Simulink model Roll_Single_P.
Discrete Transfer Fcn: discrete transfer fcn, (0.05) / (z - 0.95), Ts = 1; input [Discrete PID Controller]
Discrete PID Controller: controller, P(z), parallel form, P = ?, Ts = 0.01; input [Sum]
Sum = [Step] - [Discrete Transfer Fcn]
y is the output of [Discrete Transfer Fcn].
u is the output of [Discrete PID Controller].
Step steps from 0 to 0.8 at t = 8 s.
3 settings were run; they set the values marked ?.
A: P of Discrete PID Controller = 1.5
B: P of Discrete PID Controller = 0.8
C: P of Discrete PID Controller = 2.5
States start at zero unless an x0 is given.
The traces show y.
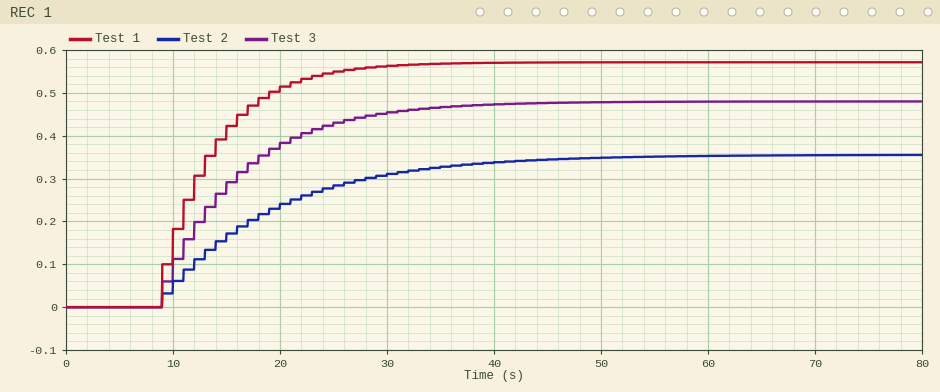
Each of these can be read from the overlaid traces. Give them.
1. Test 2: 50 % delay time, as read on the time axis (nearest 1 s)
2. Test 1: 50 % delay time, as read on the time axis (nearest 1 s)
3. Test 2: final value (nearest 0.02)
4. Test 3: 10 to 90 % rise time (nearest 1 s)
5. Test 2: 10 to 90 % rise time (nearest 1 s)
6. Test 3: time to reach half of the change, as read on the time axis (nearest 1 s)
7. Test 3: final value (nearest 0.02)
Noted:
16 s
12 s
0.36
17 s
23 s
14 s
0.48
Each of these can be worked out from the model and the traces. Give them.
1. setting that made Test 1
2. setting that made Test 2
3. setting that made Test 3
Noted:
C
B
A
